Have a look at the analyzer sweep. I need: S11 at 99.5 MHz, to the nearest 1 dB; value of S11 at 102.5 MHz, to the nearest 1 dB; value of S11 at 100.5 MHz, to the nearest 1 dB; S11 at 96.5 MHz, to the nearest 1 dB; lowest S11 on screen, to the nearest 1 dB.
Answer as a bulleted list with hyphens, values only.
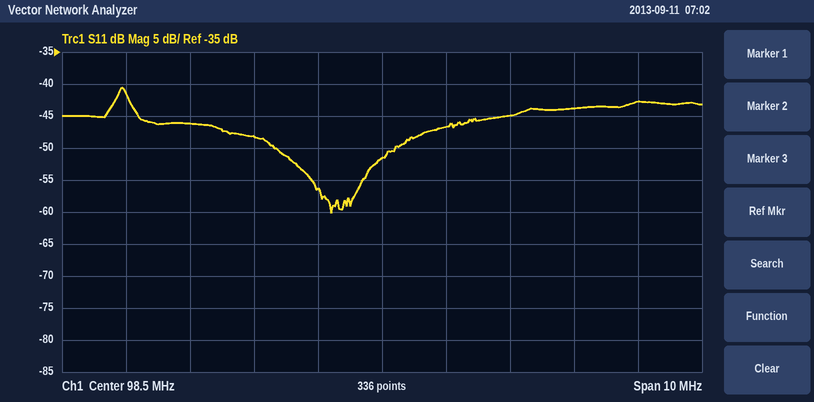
- -47 dB
- -43 dB
- -45 dB
- -48 dB
- -60 dB
